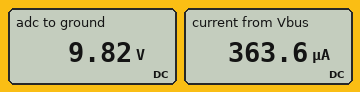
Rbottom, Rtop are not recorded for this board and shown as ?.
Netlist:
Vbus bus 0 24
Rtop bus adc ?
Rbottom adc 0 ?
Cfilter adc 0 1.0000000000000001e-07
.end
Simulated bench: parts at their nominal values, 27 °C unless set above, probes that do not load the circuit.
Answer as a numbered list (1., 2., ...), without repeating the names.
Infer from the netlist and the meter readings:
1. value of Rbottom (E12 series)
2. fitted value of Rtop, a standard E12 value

1. 27 kΩ
2. 39 kΩ
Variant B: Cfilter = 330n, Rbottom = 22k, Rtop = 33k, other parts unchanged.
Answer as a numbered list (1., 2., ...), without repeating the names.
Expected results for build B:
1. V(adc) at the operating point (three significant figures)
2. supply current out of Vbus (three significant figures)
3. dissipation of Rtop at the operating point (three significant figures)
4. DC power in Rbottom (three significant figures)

1. 9.60 V
2. 436 µA
3. 6.28 mW
4. 4.19 mW
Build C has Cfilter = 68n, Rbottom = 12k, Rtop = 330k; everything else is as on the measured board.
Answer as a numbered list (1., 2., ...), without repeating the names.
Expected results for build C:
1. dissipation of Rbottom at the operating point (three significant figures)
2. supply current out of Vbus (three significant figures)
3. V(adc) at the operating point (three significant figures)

1. 59.1 µW
2. 70.2 µA
3. 842 mV
